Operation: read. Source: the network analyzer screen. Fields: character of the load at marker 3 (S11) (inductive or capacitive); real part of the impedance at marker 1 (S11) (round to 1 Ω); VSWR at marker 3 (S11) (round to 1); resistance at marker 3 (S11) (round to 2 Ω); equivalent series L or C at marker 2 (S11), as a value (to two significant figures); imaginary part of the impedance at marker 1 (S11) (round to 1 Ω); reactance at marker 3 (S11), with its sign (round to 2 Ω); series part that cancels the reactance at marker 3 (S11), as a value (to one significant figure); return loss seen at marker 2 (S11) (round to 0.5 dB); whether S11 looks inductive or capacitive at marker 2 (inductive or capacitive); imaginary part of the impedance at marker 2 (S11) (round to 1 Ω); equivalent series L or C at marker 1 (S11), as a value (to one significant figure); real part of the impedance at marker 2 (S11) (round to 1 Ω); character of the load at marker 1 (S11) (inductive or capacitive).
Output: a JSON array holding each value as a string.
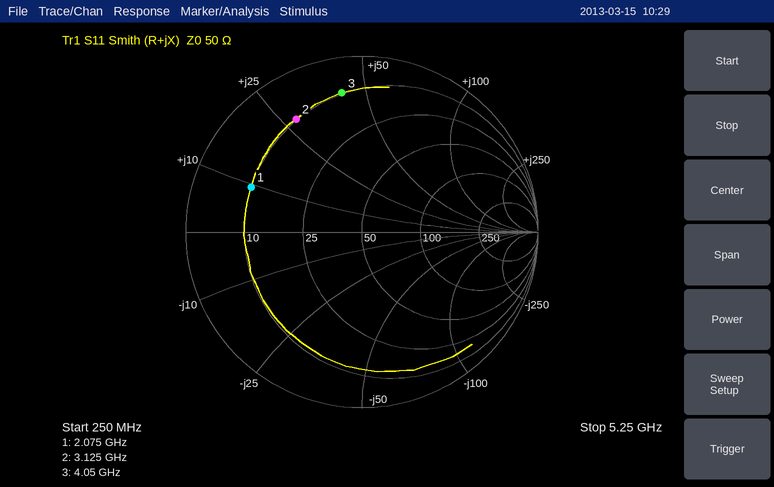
["inductive", "10 Ω", "9", "10 Ω", "1.4 nH", "+9 Ω", "+42 Ω", "900 fF", "2.5 dB", "inductive", "+28 Ω", "700 pH", "10 Ω", "inductive"]
